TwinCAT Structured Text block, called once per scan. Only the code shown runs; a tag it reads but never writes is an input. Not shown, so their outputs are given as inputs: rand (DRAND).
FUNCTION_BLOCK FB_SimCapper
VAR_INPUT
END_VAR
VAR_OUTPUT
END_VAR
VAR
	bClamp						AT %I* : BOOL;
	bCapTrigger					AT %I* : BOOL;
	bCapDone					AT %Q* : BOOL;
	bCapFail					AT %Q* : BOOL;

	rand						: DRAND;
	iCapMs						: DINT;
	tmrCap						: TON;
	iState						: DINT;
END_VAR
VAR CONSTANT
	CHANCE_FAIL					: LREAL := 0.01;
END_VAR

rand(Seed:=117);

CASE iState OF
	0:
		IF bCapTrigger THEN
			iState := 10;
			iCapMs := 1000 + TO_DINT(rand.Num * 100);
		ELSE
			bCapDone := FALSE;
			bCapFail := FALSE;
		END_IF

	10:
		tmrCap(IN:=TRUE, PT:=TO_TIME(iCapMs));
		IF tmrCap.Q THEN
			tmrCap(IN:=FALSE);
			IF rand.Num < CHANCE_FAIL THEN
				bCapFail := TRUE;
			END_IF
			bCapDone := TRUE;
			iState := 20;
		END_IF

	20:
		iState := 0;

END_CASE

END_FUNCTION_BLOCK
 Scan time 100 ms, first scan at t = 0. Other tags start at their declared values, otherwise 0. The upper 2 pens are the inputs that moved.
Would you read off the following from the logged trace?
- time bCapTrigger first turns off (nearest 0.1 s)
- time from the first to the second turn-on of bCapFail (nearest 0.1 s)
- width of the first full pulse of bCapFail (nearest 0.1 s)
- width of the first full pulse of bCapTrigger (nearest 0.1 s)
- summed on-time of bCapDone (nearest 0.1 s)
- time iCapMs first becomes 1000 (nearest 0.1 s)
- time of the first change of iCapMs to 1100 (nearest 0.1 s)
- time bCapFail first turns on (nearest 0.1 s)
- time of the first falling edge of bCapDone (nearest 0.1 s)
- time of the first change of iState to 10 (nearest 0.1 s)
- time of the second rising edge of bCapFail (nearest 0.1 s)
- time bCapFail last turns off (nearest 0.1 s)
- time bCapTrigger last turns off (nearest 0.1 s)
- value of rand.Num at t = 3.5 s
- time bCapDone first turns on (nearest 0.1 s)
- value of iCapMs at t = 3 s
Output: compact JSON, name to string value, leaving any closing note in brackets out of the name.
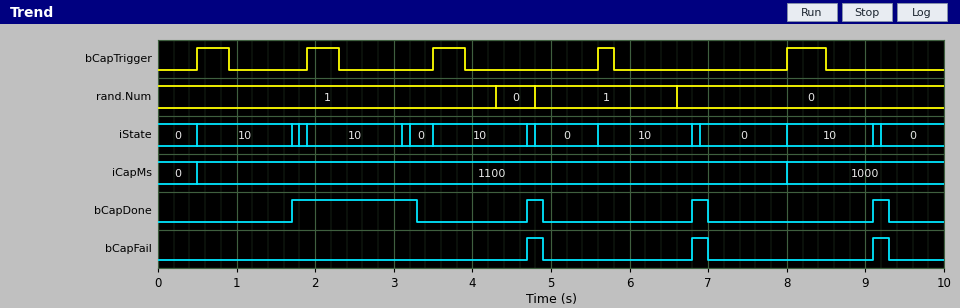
{"time bCapTrigger first turns off": "0.9 s", "time from the first to the second turn-on of bCapFail": "2.1 s", "width of the first full pulse of bCapFail": "0.2 s", "width of the first full pulse of bCapTrigger": "0.4 s", "summed on-time of bCapDone": "2.2 s", "time iCapMs first becomes 1000": "8.0 s", "time of the first change of iCapMs to 1100": "0.5 s", "time bCapFail first turns on": "4.7 s", "time of the first falling edge of bCapDone": "3.3 s", "time of the first change of iState to 10": "0.5 s", "time of the second rising edge of bCapFail": "6.8 s", "time bCapFail last turns off": "9.3 s", "time bCapTrigger last turns off": "8.5 s", "value of rand.Num at t = 3.5 s": "1", "time bCapDone first turns on": "1.7 s", "value of iCapMs at t = 3 s": "1100"}
